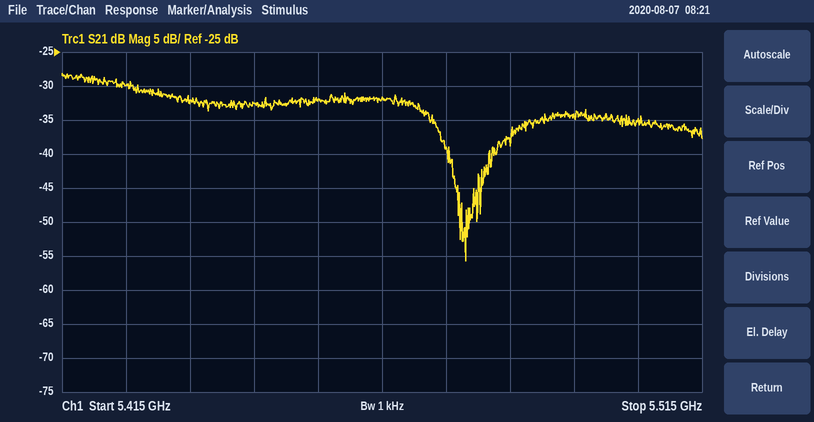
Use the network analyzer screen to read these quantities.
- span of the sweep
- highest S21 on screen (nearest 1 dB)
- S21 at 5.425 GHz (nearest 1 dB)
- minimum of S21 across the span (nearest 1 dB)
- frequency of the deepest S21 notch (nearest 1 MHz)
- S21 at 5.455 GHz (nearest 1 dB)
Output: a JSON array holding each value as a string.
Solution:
["100 MHz", "-28 dB", "-30 dB", "-56 dB", "5.478 GHz", "-32 dB"]
